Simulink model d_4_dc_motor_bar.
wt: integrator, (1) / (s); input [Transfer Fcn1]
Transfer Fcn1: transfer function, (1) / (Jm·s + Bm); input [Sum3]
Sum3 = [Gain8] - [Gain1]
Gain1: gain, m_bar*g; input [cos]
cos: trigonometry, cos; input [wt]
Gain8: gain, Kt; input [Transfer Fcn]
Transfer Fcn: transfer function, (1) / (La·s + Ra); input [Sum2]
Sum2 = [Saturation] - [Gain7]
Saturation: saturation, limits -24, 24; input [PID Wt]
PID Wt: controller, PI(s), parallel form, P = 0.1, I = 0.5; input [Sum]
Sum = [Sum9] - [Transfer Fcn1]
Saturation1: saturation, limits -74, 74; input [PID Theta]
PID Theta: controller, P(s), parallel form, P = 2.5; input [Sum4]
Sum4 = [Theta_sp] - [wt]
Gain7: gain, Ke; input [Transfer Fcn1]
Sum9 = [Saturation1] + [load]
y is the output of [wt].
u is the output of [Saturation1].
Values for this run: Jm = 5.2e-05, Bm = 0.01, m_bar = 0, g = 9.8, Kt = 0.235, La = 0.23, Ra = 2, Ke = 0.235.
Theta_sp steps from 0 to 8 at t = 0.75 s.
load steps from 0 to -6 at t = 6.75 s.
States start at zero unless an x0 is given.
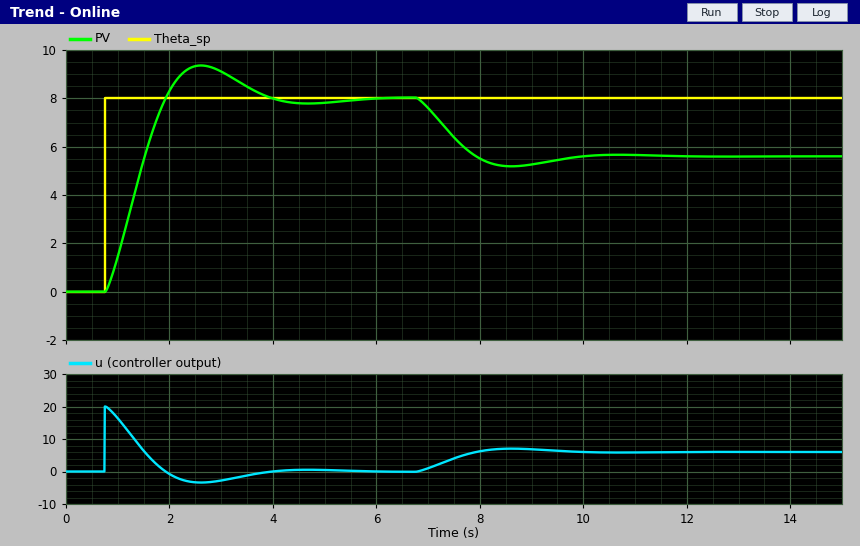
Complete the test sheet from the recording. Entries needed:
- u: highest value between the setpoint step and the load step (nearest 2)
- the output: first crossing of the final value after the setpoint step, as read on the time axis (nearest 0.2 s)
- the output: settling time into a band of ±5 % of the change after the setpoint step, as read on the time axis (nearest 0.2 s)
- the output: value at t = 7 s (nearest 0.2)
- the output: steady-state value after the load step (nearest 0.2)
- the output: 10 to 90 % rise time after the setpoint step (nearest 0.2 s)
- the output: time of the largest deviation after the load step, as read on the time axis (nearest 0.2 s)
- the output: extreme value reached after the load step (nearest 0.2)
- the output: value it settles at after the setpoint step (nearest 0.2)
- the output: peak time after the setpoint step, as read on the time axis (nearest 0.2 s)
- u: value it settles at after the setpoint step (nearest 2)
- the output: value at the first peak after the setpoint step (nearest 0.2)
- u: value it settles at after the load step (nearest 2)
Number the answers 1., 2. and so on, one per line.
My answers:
1. 20
2. 2.0 s
3. 3.6 s
4. 7.6
5. 5.6
6. 0.8 s
7. 8.6 s
8. 5.2
9. 8.0
10. 2.6 s
11. 0
12. 9.4
13. 6
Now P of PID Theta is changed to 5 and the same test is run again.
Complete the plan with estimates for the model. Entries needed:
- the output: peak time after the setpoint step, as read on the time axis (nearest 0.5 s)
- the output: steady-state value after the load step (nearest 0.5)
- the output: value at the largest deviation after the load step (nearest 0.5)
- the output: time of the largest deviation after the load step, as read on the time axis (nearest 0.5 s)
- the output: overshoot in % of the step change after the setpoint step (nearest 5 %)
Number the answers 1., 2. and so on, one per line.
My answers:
1. 2.0 s
2. 7.0
3. 6.5
4. 8.0 s
5. 20 %
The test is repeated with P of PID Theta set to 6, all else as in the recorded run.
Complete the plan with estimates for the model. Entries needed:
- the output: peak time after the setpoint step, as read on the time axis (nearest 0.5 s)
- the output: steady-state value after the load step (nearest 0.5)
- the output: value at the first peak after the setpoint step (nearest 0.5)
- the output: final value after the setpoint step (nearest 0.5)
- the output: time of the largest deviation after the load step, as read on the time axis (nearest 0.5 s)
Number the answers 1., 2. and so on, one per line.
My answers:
1. 2.0 s
2. 7.0
3. 10.0
4. 8.0
5. 8.0 s
